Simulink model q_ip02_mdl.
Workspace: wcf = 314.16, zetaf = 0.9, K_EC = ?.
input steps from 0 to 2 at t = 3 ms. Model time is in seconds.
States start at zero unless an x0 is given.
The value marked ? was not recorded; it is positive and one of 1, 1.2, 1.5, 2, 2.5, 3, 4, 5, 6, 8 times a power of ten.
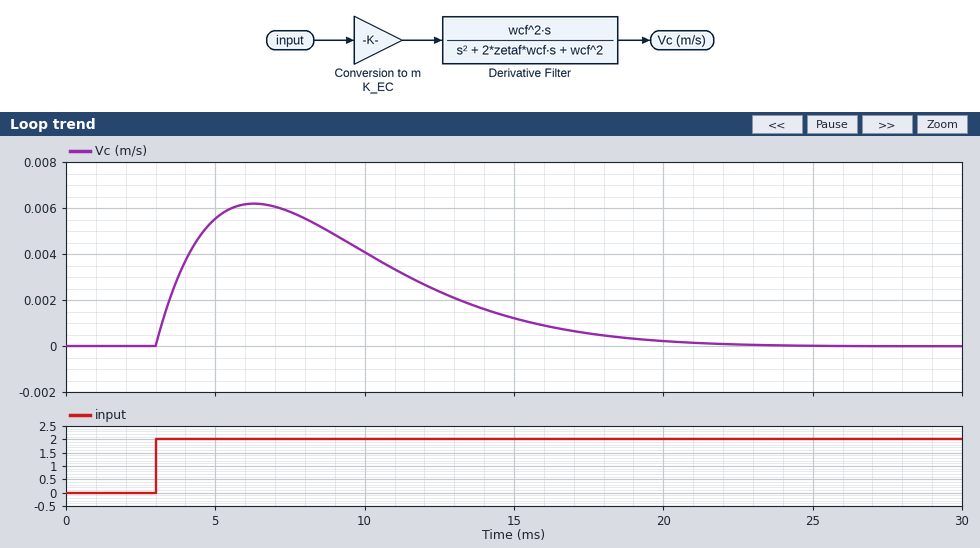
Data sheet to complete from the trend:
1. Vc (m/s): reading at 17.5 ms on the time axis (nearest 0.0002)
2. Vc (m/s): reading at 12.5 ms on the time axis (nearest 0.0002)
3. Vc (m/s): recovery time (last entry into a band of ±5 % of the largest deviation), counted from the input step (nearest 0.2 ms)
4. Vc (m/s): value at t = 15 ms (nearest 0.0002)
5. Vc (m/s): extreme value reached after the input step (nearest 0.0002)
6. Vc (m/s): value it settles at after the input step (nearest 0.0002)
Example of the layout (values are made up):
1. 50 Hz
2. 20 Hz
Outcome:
1. 0.0006
2. 0.0024
3. 16.0 ms
4. 0.0012
5. 0.0062
6. 0.0000
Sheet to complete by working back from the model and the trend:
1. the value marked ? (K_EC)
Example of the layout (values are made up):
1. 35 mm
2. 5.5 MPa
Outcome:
1. 2.5e-05
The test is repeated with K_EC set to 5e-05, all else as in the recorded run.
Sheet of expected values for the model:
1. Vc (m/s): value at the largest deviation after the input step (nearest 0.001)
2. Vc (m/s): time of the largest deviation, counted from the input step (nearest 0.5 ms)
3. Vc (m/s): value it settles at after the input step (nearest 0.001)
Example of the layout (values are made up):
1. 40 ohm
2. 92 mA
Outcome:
1. 0.012
2. 3.5 ms
3. 0.000
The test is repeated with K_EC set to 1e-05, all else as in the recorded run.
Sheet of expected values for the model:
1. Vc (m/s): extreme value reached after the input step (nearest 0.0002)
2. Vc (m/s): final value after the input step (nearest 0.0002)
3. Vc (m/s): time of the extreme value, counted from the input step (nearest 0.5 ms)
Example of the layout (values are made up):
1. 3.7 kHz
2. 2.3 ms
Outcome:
1. 0.0024
2. 0.0000
3. 3.5 ms
